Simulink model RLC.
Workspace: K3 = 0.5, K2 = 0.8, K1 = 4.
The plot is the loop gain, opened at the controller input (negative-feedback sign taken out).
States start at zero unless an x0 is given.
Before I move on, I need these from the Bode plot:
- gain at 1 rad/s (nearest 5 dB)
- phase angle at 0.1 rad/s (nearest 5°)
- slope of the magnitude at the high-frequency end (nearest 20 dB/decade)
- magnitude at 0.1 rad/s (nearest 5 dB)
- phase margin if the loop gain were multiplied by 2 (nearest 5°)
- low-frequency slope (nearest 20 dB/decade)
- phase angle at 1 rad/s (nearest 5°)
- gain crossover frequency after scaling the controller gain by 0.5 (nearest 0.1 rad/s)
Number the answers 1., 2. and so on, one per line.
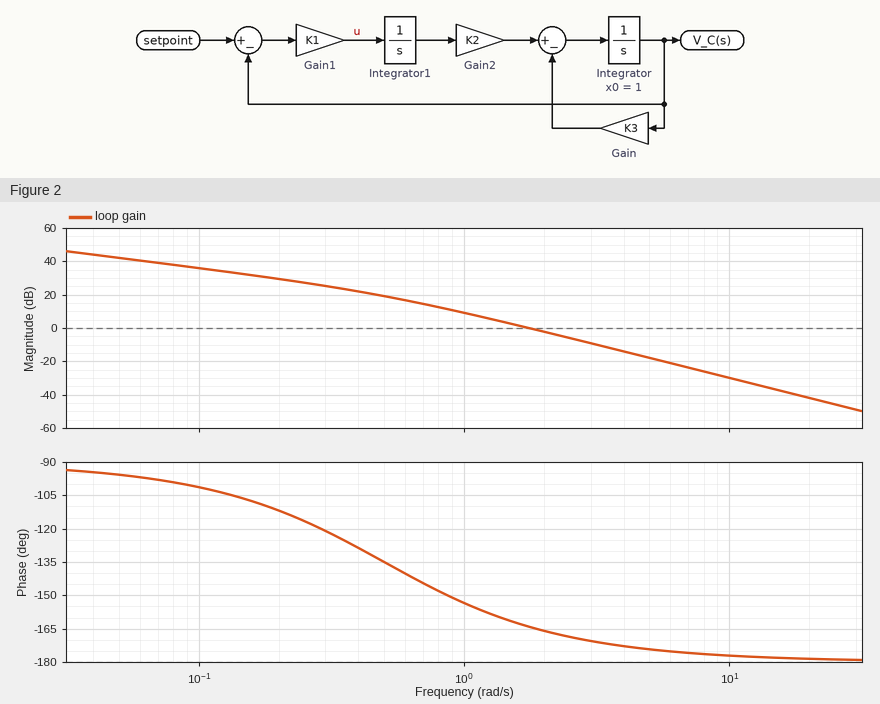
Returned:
1. 10 dB
2. -100°
3. -40 dB/decade
4. 35 dB
5. 10°
6. -20 dB/decade
7. -155°
8. 1.2 rad/s
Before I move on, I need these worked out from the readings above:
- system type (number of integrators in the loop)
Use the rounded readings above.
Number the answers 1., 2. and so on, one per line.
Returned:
1. 1
